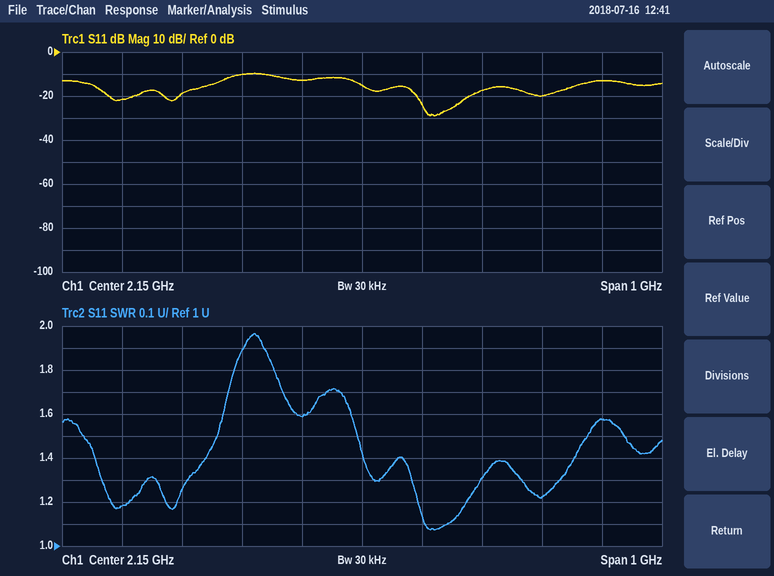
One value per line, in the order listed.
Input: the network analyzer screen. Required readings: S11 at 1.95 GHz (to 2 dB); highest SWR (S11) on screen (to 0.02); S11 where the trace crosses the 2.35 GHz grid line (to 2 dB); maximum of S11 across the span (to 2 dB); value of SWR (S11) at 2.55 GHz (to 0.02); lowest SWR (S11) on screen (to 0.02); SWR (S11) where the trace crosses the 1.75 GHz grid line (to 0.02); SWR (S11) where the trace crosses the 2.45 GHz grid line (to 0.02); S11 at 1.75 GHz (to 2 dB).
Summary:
-10 dB
1.96
-18 dB
-10 dB
1.58
1.08
1.18
1.22
-22 dB
